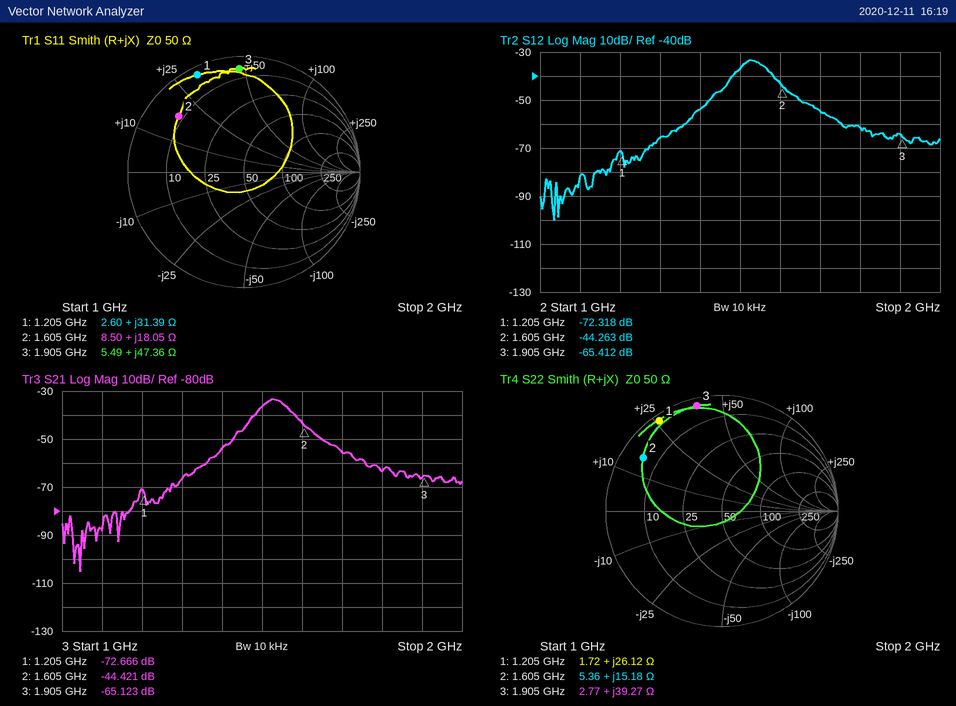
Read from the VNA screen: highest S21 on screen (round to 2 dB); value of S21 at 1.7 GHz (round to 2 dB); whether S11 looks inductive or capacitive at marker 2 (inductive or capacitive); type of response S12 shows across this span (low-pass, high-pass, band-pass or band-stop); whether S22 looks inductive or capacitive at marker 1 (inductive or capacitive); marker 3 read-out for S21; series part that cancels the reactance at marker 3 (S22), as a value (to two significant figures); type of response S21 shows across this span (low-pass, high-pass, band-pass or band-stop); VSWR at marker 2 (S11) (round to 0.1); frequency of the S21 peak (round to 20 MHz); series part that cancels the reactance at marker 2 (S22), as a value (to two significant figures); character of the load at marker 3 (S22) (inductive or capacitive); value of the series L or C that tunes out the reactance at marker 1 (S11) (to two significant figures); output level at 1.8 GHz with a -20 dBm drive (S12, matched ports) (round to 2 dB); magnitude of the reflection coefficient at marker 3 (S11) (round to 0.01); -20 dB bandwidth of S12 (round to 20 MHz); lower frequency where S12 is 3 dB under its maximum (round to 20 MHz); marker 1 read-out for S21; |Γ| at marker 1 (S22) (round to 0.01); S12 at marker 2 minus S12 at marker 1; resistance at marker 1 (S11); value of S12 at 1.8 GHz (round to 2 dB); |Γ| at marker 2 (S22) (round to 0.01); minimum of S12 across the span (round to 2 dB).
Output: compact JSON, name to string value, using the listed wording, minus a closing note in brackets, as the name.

{"highest S21 on screen": "-34 dB", "value of S21 at 1.7 GHz": "-56 dB", "whether S11 looks inductive or capacitive at marker 2": "inductive", "type of response S12 shows across this span": "band-pass", "whether S22 looks inductive or capacitive at marker 1": "inductive", "marker 3 read-out for S21": "-65.123 dB", "series part that cancels the reactance at marker 3 (S22), as a value": "2.1 pF", "type of response S21 shows across this span": "band-pass", "VSWR at marker 2 (S11)": "6.7", "frequency of the S21 peak": "1.52 GHz", "series part that cancels the reactance at marker 2 (S22), as a value": "6.5 pF", "character of the load at marker 3 (S22)": "inductive", "value of the series L or C that tunes out the reactance at marker 1 (S11)": "4.2 pF", "output level at 1.8 GHz with a -20 dBm drive (S12, matched ports)": "-82 dBm", "magnitude of the reflection coefficient at marker 3 (S11)": "0.89", "-20 dB bandwidth of S12": "280 MHz", "lower frequency where S12 is 3 dB under its maximum": "1.50 GHz", "marker 1 read-out for S21": "-72.666 dB", "|Γ| at marker 1 (S22)": "0.95", "S12 at marker 2 minus S12 at marker 1": "28.055 dB", "resistance at marker 1": "2.60 Ω", "value of S12 at 1.8 GHz": "-62 dB", "|Γ| at marker 2 (S22)": "0.82", "minimum of S12 across the span": "-100 dB"}
